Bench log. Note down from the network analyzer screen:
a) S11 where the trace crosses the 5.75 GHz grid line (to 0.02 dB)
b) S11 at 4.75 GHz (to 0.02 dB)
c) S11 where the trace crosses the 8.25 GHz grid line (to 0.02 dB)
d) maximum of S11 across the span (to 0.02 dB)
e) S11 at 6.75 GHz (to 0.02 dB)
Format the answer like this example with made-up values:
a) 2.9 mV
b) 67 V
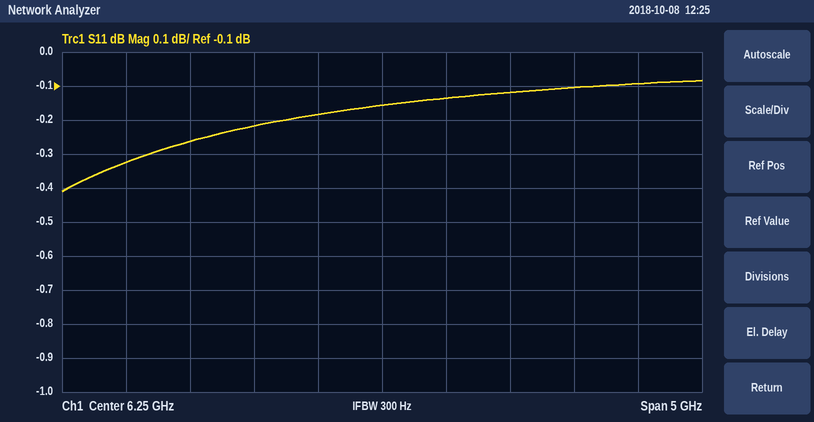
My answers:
a) -0.18 dB
b) -0.26 dB
c) -0.10 dB
d) -0.08 dB
e) -0.14 dB
